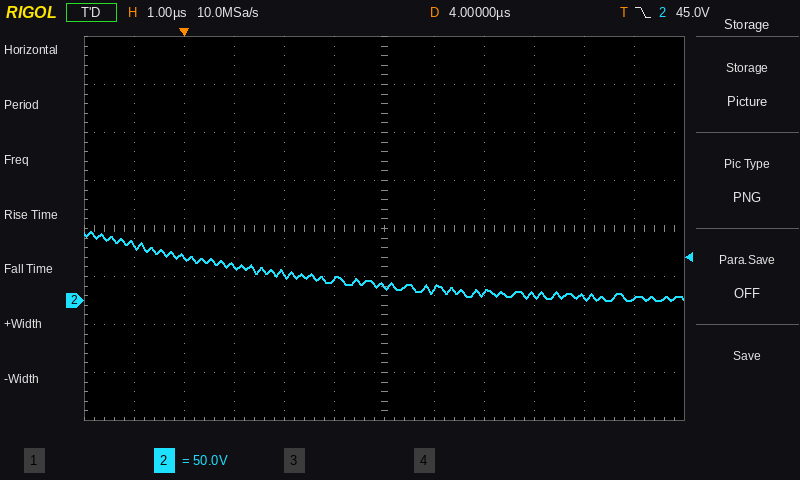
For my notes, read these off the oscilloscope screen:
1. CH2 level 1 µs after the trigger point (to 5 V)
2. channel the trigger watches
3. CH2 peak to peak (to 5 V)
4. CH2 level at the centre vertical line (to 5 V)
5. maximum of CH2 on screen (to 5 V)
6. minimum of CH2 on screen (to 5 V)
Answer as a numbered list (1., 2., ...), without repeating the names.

1. 35 V
2. CH2
3. 70 V
4. 15 V
5. 70 V
6. 0 V
